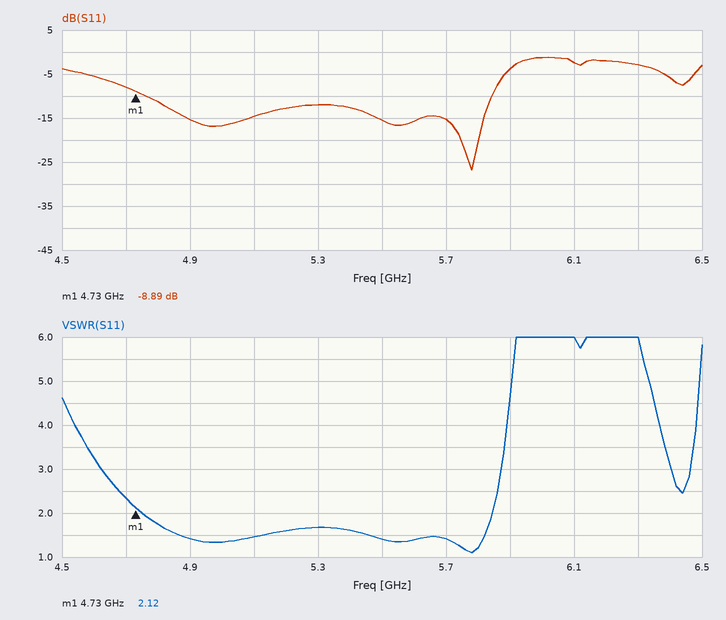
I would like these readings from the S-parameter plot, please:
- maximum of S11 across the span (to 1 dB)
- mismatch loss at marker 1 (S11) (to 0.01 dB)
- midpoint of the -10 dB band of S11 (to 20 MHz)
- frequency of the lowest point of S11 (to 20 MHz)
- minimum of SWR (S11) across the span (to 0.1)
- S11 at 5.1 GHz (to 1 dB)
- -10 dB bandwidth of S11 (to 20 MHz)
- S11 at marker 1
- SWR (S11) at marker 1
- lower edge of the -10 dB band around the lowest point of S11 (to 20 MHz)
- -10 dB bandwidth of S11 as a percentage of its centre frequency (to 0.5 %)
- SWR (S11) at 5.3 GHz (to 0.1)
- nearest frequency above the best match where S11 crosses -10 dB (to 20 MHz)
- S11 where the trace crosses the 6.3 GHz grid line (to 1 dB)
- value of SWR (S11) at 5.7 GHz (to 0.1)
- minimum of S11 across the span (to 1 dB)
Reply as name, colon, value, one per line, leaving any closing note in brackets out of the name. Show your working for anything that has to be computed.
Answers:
maximum of S11 across the span: -1 dB
mismatch loss at marker 1 (S11): −10 log10(1 − 10^(-8.89/10)) ≈ 0.60 dB
midpoint of the -10 dB band of S11: 5.30 GHz
frequency of the lowest point of S11: 5.78 GHz
minimum of SWR (S11) across the span: 1.1
S11 at 5.1 GHz: -15 dB
-10 dB bandwidth of S11: 5.84 GHz − 4.76 GHz = 1.08 GHz
S11 at marker 1: -8.89 dB
SWR (S11) at marker 1: 2.12
lower edge of the -10 dB band around the lowest point of S11: 4.76 GHz
-10 dB bandwidth of S11 as a percentage of its centre frequency: 1.08 GHz / 5.3 GHz ≈ 20.4 %, so 20.5 % to the nearest 0.5 %
SWR (S11) at 5.3 GHz: 1.7
nearest frequency above the best match where S11 crosses -10 dB: 5.84 GHz
S11 where the trace crosses the 6.3 GHz grid line: -3 dB
value of SWR (S11) at 5.7 GHz: 1.4
minimum of S11 across the span: -27 dB
